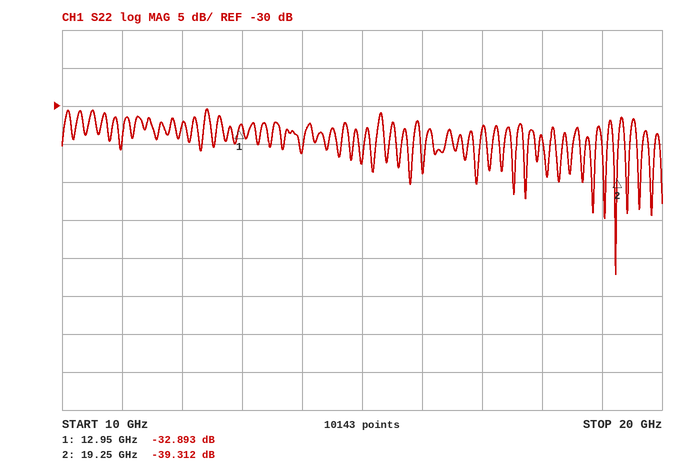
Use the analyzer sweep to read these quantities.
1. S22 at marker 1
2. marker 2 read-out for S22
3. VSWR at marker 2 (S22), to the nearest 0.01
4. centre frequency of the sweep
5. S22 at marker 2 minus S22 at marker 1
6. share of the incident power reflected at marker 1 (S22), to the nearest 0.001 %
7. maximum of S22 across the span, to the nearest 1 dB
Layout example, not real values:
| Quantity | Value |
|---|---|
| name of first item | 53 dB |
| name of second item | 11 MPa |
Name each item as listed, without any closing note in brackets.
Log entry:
| Quantity | Value |
|---|---|
| S22 at marker 1 | -32.893 dB |
| marker 2 read-out for S22 | -39.312 dB |
| VSWR at marker 2 (S22), to the nearest 0.01 | 1.02 |
| centre frequency of the sweep | 15 GHz |
| S22 at marker 2 minus S22 at marker 1 | -6.419 dB |
| share of the incident power reflected at marker 1 (S22), to the nearest 0.001 % | 0.051 % |
| maximum of S22 across the span, to the nearest 1 dB | -30 dB |
